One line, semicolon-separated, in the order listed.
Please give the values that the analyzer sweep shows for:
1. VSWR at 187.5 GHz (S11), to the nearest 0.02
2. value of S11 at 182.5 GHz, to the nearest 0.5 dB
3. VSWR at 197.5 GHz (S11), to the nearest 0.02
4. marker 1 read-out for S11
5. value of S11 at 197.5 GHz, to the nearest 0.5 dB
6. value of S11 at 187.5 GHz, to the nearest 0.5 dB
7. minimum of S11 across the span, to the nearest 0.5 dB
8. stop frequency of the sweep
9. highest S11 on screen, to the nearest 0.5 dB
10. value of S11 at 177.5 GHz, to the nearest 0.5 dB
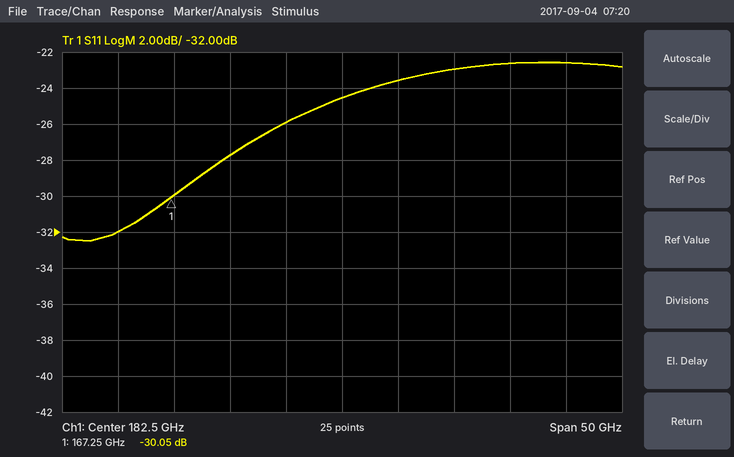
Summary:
1.14; -24.5 dB; 1.16; -30.05 dB; -22.5 dB; -23.5 dB; -32.5 dB; 207.5 GHz; -22.5 dB; -26.0 dB
